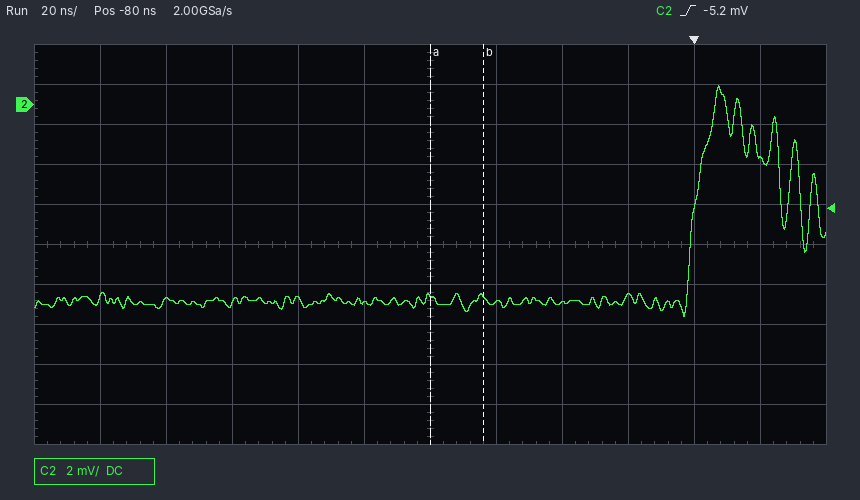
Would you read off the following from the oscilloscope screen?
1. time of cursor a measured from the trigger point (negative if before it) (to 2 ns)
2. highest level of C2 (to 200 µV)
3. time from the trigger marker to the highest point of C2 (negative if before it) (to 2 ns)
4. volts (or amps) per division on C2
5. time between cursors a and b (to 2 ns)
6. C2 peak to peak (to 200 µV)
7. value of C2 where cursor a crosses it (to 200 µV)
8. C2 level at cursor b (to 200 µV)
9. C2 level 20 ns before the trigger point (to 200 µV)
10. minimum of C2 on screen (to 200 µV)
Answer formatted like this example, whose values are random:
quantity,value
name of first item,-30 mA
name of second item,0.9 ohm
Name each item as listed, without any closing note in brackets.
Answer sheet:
quantity,value
time of cursor a measured from the trigger point (negative if before it),-80 ns
highest level of C2,1.0 mV
time from the trigger marker to the highest point of C2 (negative if before it),+8 ns
volts (or amps) per division on C2,2 mV
time between cursors a and b,16 ns
C2 peak to peak,11.6 mV
value of C2 where cursor a crosses it,-9.6 mV
C2 level at cursor b,-9.6 mV
C2 level 20 ns before the trigger point,-9.6 mV
minimum of C2 on screen,-10.6 mV
